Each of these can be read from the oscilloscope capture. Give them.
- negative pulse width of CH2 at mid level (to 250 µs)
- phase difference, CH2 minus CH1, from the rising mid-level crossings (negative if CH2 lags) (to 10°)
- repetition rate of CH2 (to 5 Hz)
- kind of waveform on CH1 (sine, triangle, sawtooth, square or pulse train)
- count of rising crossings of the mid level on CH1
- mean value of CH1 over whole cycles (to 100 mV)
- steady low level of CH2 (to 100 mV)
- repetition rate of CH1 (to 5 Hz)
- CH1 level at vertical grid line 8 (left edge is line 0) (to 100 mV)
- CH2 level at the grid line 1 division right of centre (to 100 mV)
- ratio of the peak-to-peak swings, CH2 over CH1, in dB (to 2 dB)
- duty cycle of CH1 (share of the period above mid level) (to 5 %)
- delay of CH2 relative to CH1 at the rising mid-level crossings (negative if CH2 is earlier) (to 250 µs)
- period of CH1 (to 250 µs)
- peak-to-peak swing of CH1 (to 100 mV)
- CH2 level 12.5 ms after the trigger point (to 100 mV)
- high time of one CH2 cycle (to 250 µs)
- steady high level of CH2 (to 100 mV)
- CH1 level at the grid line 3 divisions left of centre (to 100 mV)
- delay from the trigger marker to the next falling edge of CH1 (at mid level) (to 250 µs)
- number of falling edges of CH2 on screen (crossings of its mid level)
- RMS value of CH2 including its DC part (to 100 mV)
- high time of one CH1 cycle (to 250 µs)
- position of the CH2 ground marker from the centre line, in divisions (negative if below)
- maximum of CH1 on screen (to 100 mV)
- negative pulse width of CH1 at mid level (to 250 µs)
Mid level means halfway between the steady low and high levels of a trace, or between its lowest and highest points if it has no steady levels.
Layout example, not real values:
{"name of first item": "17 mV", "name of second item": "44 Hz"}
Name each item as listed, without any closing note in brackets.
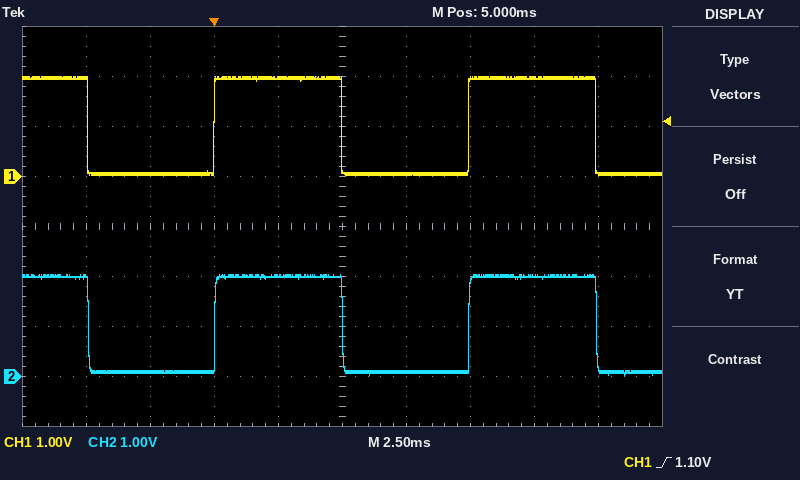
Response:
{"negative pulse width of CH2 at mid level": "5.00 ms", "phase difference, CH2 minus CH1, from the rising mid-level crossings (negative if CH2 lags)": "0°", "repetition rate of CH2": "100 Hz", "kind of waveform on CH1": "square", "count of rising crossings of the mid level on CH1": "2", "mean value of CH1 over whole cycles": "1.0 V", "steady low level of CH2": "100 mV", "repetition rate of CH1": "100 Hz", "CH1 level at vertical grid line 8 (left edge is line 0)": "2.0 V", "CH2 level at the grid line 1 division right of centre": "100 mV", "ratio of the peak-to-peak swings, CH2 over CH1, in dB": "0 dB", "duty cycle of CH1 (share of the period above mid level)": "50 %", "delay of CH2 relative to CH1 at the rising mid-level crossings (negative if CH2 is earlier)": "0.00 ms", "period of CH1": "10.00 ms", "peak-to-peak swing of CH1": "2.0 V", "CH2 level 12.5 ms after the trigger point": "2.0 V", "high time of one CH2 cycle": "5.00 ms", "steady high level of CH2": "2.0 V", "CH1 level at the grid line 3 divisions left of centre": "100 mV", "delay from the trigger marker to the next falling edge of CH1 (at mid level)": "5.00 ms", "number of falling edges of CH2 on screen": "3", "RMS value of CH2 including its DC part": "1.4 V", "high time of one CH1 cycle": "5.00 ms", "position of the CH2 ground marker from the centre line, in divisions": "-3.0 div", "maximum of CH1 on screen": "2.0 V", "negative pulse width of CH1 at mid level": "5.00 ms"}
